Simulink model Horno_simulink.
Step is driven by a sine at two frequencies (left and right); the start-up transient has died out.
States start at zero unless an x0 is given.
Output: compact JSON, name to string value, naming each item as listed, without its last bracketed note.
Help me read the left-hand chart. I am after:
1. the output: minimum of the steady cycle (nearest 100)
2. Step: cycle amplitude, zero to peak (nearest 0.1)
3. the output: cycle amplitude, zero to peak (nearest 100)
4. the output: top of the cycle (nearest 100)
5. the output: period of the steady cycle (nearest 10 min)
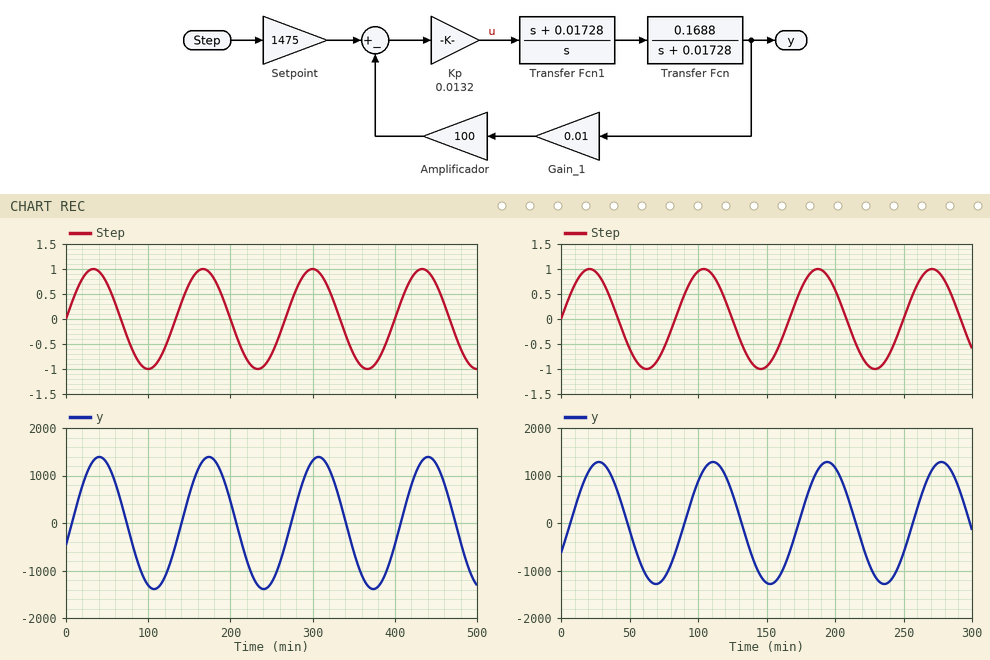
{"the output: minimum of the steady cycle": "-1400", "Step: cycle amplitude, zero to peak": "1.0", "the output: cycle amplitude, zero to peak": "1400", "the output: top of the cycle": "1400", "the output: period of the steady cycle": "130 min"}
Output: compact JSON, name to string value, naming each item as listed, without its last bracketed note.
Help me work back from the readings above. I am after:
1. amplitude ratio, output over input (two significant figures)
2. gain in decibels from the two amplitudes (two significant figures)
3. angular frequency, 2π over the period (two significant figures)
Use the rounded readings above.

{"amplitude ratio, output over input": "1400", "gain in decibels from the two amplitudes": "63 dB", "angular frequency, 2π over the period": "0.048 rad/min"}
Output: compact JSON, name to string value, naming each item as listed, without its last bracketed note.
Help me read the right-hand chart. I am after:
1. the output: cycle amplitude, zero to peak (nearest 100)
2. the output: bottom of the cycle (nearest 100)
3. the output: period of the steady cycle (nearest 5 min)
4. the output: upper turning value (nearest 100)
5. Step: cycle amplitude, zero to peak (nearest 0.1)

{"the output: cycle amplitude, zero to peak": "1300", "the output: bottom of the cycle": "-1300", "the output: period of the steady cycle": "85 min", "the output: upper turning value": "1300", "Step: cycle amplitude, zero to peak": "1.0"}
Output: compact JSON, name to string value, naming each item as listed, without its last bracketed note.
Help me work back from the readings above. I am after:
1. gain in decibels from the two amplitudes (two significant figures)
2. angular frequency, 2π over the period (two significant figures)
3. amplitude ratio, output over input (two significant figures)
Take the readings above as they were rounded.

{"gain in decibels from the two amplitudes": "62 dB", "angular frequency, 2π over the period": "0.074 rad/min", "amplitude ratio, output over input": "1300"}
